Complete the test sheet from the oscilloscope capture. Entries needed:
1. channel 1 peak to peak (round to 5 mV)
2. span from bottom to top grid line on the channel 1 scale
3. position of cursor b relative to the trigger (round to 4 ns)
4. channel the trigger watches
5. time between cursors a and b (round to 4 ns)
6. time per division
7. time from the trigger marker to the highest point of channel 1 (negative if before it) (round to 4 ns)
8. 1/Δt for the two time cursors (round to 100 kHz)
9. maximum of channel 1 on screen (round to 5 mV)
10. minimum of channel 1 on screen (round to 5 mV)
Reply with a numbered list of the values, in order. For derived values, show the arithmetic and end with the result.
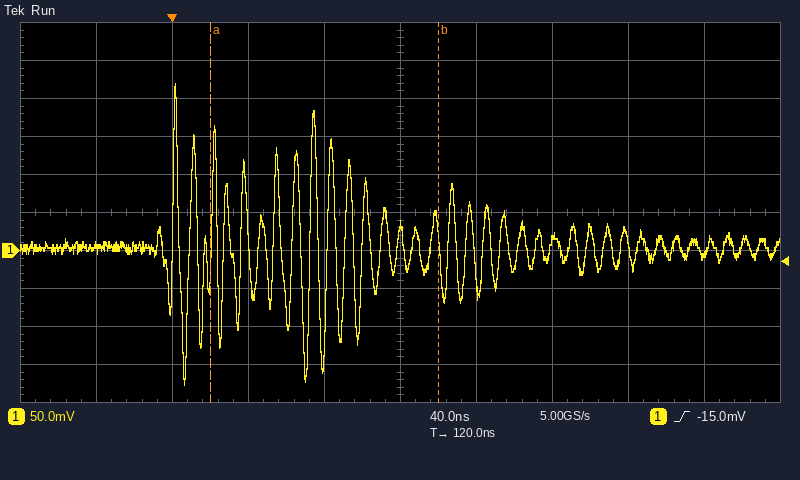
1. 220 mV − (-175 mV) = 395 mV
2. 500 mV
3. +140 ns
4. channel 1
5. 120 ns
6. 40 ns
7. 0 ns
8. 1 / 120 ns ≈ 8.3 MHz
9. 220 mV
10. -175 mV
